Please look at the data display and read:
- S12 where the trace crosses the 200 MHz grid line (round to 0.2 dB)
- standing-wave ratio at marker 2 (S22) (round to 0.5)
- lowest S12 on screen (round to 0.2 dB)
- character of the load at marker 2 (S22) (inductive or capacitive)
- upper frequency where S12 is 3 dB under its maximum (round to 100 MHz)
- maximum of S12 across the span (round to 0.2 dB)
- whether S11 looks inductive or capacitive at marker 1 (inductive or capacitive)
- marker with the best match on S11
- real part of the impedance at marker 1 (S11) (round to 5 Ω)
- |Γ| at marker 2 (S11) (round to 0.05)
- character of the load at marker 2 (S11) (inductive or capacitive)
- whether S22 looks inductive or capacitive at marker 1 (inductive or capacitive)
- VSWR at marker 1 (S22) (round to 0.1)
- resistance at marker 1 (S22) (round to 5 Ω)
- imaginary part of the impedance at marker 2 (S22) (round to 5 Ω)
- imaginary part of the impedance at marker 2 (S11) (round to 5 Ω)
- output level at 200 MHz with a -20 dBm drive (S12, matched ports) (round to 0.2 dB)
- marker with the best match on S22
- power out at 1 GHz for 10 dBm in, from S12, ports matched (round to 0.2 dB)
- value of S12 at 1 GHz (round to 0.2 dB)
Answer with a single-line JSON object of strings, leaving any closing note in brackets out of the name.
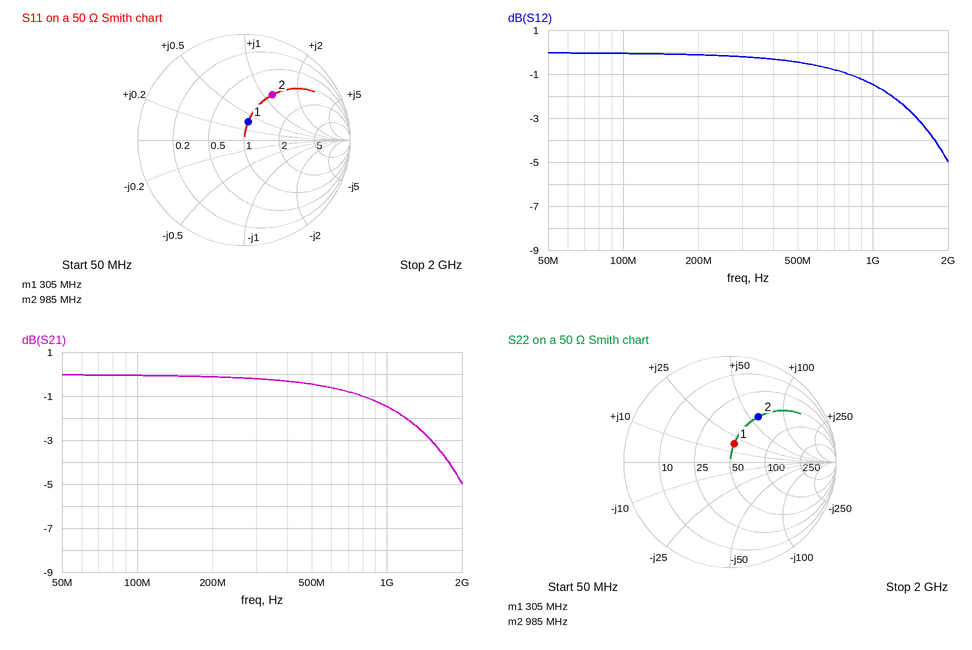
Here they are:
{"S12 where the trace crosses the 200 MHz grid line": "-0.2 dB", "standing-wave ratio at marker 2 (S22)": "3.0", "lowest S12 on screen": "-5.0 dB", "character of the load at marker 2 (S22)": "inductive", "upper frequency where S12 is 3 dB under its maximum": "1.5 GHz", "maximum of S12 across the span": "0.0 dB", "whether S11 looks inductive or capacitive at marker 1": "inductive", "marker with the best match on S11": "marker 1", "real part of the impedance at marker 1 (S11)": "50 Ω", "|Γ| at marker 2 (S11)": "0.50", "character of the load at marker 2 (S11)": "inductive", "whether S22 looks inductive or capacitive at marker 1": "inductive", "VSWR at marker 1 (S22)": "1.4", "resistance at marker 1 (S22)": "50 Ω", "imaginary part of the impedance at marker 2 (S22)": "+60 Ω", "imaginary part of the impedance at marker 2 (S11)": "+60 Ω", "output level at 200 MHz with a -20 dBm drive (S12, matched ports)": "-20.2 dBm", "marker with the best match on S22": "marker 1", "power out at 1 GHz for 10 dBm in, from S12, ports matched": "8.6 dBm", "value of S12 at 1 GHz": "-1.4 dB"}
